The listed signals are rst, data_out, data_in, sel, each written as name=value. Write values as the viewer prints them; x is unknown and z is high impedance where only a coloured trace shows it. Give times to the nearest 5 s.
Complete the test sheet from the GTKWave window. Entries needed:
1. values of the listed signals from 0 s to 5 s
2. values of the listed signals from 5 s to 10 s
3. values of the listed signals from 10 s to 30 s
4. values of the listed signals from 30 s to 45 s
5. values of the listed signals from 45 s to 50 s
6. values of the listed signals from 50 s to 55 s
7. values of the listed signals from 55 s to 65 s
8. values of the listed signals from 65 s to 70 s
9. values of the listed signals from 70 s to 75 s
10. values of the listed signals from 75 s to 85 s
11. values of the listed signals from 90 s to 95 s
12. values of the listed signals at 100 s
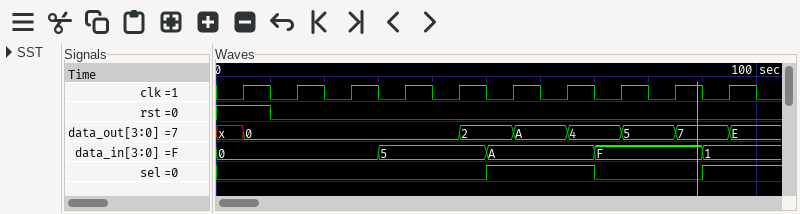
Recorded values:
rst=1, data_out=x, data_in=0, sel=0
rst=1, data_out=0, data_in=0, sel=0
rst=0, data_out=0, data_in=0, sel=0
rst=0, data_out=0, data_in=5, sel=0
rst=0, data_out=2, data_in=5, sel=0
rst=0, data_out=2, data_in=A, sel=1
rst=0, data_out=A, data_in=A, sel=1
rst=0, data_out=4, data_in=A, sel=1
rst=0, data_out=4, data_in=F, sel=0
rst=0, data_out=5, data_in=F, sel=0
rst=0, data_out=7, data_in=1, sel=1
rst=0, data_out=E, data_in=1, sel=1
